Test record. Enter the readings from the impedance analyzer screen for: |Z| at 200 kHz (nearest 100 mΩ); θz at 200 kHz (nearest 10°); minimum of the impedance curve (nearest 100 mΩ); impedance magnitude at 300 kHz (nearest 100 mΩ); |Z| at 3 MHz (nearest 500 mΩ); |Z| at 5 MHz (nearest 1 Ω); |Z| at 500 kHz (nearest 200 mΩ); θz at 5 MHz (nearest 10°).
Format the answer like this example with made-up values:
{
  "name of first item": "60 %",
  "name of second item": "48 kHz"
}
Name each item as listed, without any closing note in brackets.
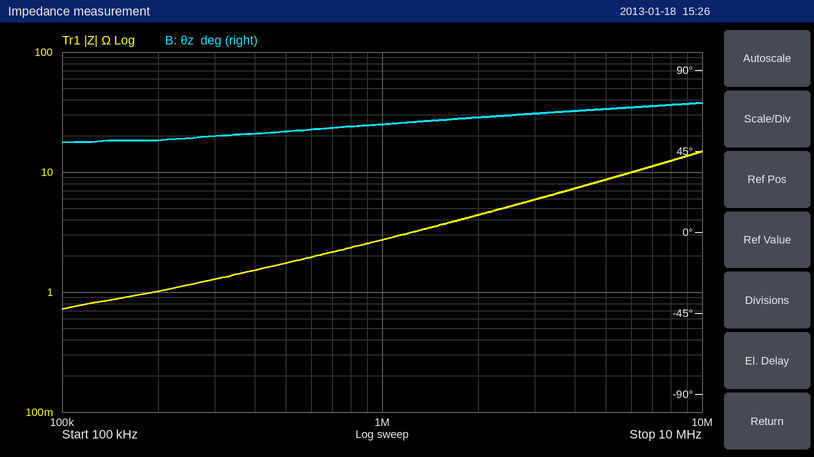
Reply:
{
  "|Z| at 200 kHz": "1.0 Ω",
  "θz at 200 kHz": "50°",
  "minimum of the impedance curve": "700 mΩ",
  "impedance magnitude at 300 kHz": "1.3 Ω",
  "|Z| at 3 MHz": "6.0 Ω",
  "|Z| at 5 MHz": "9 Ω",
  "|Z| at 500 kHz": "1.8 Ω",
  "θz at 5 MHz": "70°"
}
